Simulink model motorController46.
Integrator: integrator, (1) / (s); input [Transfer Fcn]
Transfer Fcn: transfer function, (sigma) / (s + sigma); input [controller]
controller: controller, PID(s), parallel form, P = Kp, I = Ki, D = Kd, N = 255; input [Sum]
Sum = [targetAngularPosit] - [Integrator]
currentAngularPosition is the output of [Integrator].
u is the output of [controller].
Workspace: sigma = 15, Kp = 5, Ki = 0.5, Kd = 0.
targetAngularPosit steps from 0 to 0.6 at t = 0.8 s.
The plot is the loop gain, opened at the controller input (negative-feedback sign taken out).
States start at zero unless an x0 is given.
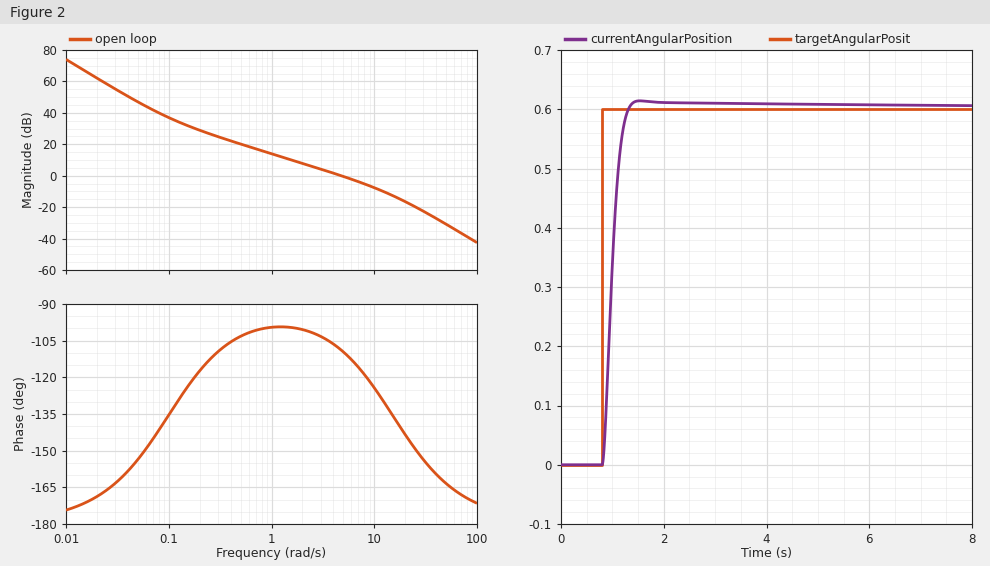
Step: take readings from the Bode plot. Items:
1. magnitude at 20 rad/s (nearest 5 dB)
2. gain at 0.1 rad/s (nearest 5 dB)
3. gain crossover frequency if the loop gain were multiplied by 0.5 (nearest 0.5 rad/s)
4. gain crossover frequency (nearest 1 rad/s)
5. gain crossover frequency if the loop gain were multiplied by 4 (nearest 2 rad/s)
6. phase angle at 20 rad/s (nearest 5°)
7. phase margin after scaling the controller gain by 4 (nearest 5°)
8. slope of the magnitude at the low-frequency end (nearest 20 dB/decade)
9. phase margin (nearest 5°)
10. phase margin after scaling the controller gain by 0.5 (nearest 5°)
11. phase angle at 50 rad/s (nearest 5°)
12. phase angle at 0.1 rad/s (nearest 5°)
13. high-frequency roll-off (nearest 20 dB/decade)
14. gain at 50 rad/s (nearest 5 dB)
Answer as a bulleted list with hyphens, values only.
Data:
- -15 dB
- 35 dB
- 2.5 rad/s
- 5 rad/s
- 14 rad/s
- -145°
- 45°
- -40 dB/decade
- 70°
- 80°
- -165°
- -135°
- -40 dB/decade
- -30 dB
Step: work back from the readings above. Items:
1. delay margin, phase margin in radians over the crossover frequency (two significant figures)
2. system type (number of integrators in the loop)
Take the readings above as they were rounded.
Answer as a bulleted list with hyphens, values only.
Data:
- 0.24 s
- 2
